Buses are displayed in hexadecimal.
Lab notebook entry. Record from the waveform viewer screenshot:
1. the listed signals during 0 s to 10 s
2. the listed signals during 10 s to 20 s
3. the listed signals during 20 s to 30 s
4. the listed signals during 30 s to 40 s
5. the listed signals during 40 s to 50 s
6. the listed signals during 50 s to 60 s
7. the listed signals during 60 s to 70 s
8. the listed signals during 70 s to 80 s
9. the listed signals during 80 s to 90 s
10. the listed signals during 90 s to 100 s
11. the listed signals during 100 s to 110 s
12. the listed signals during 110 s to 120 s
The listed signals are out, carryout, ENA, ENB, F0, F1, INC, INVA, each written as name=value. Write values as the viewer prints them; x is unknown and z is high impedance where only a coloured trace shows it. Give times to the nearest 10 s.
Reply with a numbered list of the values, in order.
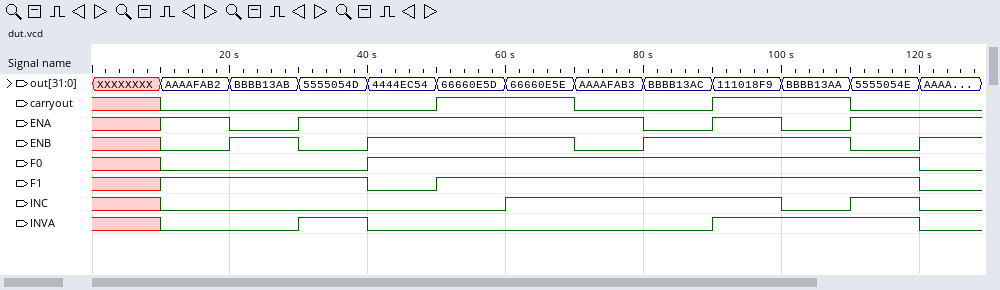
1. out=XXXXXXXX, carryout=x, ENA=x, ENB=x, F0=x, F1=x, INC=x, INVA=x
2. out=AAAAFAB2, carryout=0, ENA=1, ENB=0, F0=0, F1=1, INC=0, INVA=0
3. out=BBBB13AB, carryout=0, ENA=0, ENB=1, F0=0, F1=1, INC=0, INVA=0
4. out=5555054D, carryout=0, ENA=1, ENB=0, F0=0, F1=1, INC=0, INVA=1
5. out=4444EC54, carryout=0, ENA=1, ENB=1, F0=1, F1=0, INC=0, INVA=0
6. out=66660E5D, carryout=1, ENA=1, ENB=1, F0=1, F1=1, INC=0, INVA=0
7. out=66660E5E, carryout=1, ENA=1, ENB=1, F0=1, F1=1, INC=1, INVA=0
8. out=AAAAFAB3, carryout=0, ENA=1, ENB=0, F0=1, F1=1, INC=1, INVA=0
9. out=BBBB13AC, carryout=0, ENA=0, ENB=1, F0=1, F1=1, INC=1, INVA=0
10. out=111018F9, carryout=1, ENA=1, ENB=1, F0=1, F1=1, INC=1, INVA=1
11. out=BBBB13AA, carryout=1, ENA=0, ENB=1, F0=1, F1=1, INC=0, INVA=1
12. out=5555054E, carryout=0, ENA=1, ENB=0, F0=1, F1=1, INC=1, INVA=1
